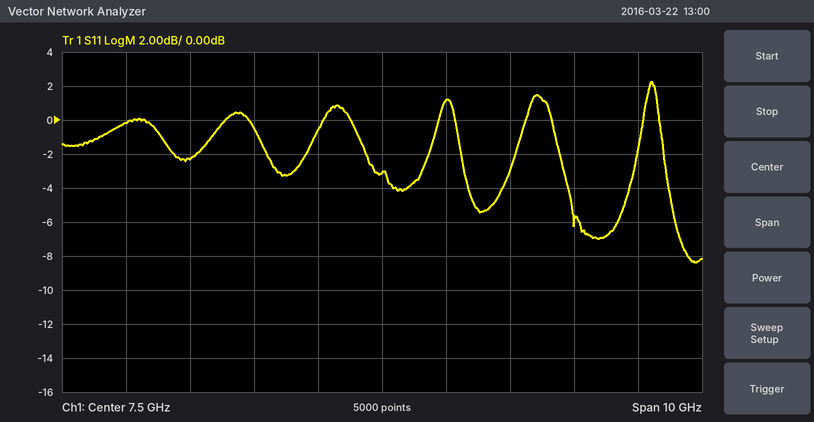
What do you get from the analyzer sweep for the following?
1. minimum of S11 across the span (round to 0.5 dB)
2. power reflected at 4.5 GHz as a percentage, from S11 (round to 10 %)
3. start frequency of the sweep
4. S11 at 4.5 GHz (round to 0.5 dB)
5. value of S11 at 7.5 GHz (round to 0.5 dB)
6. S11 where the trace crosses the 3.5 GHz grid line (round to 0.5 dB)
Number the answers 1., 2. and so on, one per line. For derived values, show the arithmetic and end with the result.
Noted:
1. -8.5 dB
2. 10^(-2.5/10) ≈ 56.2 %, so 60 % to the nearest 10 %
3. 2.5 GHz
4. -2.5 dB
5. -3.0 dB
6. 0.0 dB
